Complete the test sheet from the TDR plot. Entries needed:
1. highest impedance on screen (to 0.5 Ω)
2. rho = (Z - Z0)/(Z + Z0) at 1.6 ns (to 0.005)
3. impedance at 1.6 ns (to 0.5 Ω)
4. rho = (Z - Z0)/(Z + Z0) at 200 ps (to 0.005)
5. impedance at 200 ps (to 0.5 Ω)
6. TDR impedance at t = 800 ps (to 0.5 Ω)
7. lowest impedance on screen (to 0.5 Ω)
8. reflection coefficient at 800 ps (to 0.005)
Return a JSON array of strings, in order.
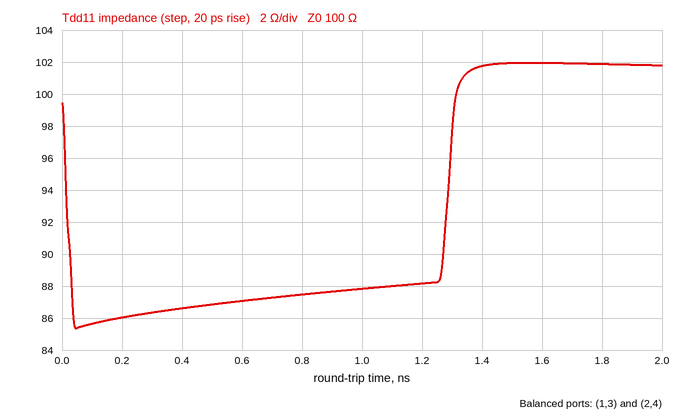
["102.0 Ω", "+0.010", "102.0 Ω", "-0.075", "86.0 Ω", "87.5 Ω", "85.5 Ω", "-0.065"]
